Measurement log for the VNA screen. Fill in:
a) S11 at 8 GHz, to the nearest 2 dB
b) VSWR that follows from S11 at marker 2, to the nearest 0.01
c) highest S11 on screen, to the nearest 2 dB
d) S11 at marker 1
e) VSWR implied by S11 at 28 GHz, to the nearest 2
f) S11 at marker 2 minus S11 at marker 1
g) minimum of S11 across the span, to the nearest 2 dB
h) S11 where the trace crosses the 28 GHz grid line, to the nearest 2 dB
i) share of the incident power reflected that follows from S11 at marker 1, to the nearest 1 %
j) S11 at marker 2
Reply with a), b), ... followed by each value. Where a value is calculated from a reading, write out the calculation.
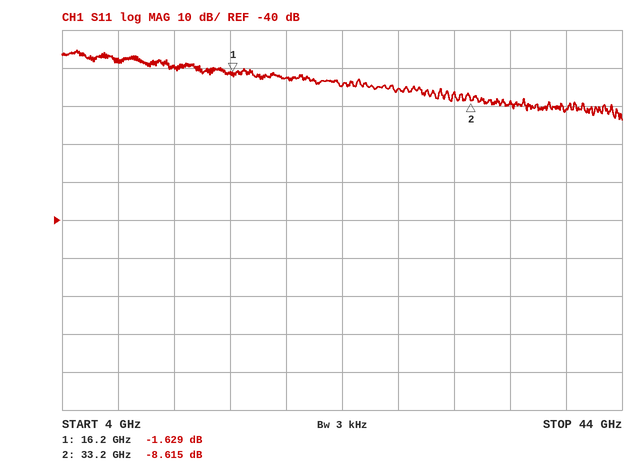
a) 2 dB
b) (1 + 0.3709)/(1 − 0.3709) ≈ 2.18
c) 4 dB
d) -1.629 dB
e) |Γ| = 10^(-6/20) = 0.5012; VSWR = (1 + 0.5012)/(1 − 0.5012) ≈ 3.01, so 4 to the nearest 2
f) -8.615 − (-1.629) = -6.986 dB
g) -14 dB
h) -6 dB
i) 10^(-1.629/10) ≈ 69 %
j) -8.615 dB
